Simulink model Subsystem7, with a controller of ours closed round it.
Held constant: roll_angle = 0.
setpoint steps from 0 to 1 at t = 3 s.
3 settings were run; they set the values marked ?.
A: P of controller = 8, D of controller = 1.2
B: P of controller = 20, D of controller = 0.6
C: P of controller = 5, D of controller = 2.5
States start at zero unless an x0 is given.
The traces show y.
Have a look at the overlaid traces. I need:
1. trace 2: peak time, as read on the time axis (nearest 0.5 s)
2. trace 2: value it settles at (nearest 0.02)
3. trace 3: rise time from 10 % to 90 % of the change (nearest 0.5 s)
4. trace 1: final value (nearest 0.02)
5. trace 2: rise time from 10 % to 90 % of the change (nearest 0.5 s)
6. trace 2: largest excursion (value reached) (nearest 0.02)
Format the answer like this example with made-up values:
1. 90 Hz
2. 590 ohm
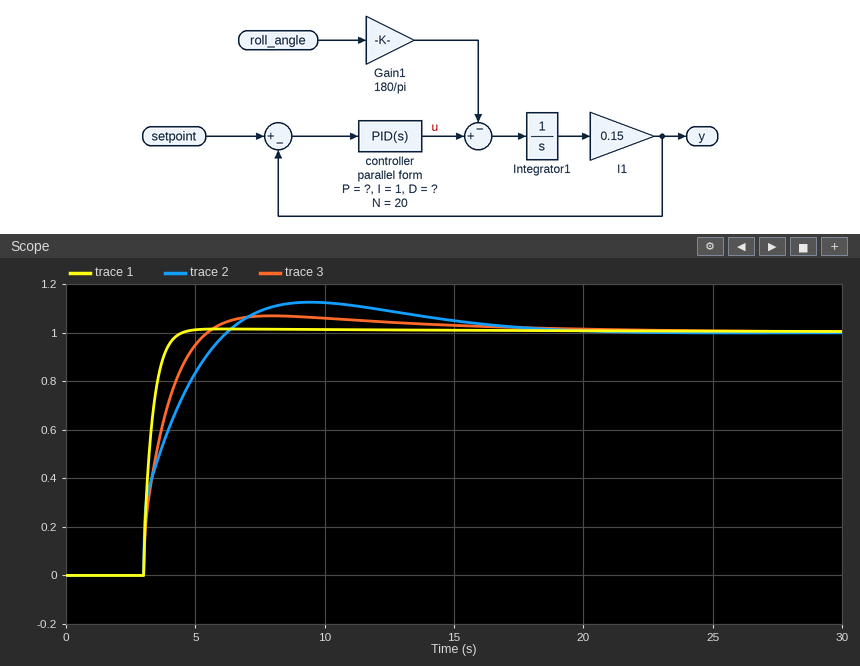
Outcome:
1. 9.5 s
2. 1.00
3. 1.5 s
4. 1.00
5. 2.5 s
6. 1.12
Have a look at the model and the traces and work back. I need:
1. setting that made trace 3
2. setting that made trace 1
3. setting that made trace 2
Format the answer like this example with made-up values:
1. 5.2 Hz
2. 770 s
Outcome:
1. A
2. B
3. C
